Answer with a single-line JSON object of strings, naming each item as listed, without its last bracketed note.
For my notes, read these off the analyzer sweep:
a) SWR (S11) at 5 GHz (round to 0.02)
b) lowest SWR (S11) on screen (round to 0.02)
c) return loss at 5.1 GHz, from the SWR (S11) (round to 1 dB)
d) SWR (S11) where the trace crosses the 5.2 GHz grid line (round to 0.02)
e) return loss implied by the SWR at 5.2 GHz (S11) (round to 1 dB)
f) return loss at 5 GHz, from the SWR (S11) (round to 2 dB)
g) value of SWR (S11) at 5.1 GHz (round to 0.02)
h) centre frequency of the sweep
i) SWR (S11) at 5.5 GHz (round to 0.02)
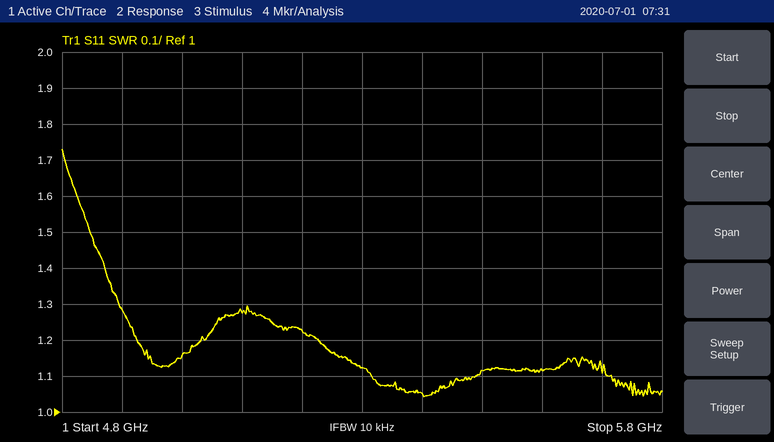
{"SWR (S11) at 5 GHz": "1.16", "lowest SWR (S11) on screen": "1.04", "return loss at 5.1 GHz, from the SWR (S11)": "18 dB", "SWR (S11) where the trace crosses the 5.2 GHz grid line": "1.22", "return loss implied by the SWR at 5.2 GHz (S11)": "20 dB", "return loss at 5 GHz, from the SWR (S11)": "22 dB", "value of SWR (S11) at 5.1 GHz": "1.28", "centre frequency of the sweep": "5.3 GHz", "SWR (S11) at 5.5 GHz": "1.12"}
